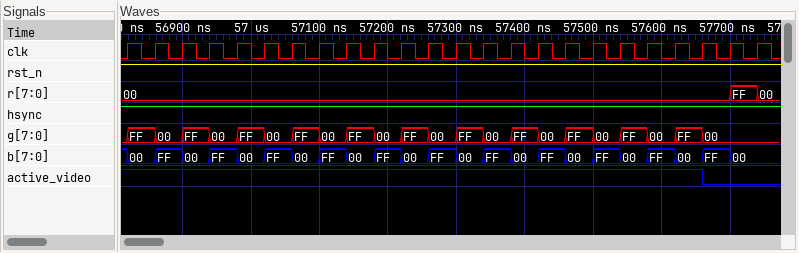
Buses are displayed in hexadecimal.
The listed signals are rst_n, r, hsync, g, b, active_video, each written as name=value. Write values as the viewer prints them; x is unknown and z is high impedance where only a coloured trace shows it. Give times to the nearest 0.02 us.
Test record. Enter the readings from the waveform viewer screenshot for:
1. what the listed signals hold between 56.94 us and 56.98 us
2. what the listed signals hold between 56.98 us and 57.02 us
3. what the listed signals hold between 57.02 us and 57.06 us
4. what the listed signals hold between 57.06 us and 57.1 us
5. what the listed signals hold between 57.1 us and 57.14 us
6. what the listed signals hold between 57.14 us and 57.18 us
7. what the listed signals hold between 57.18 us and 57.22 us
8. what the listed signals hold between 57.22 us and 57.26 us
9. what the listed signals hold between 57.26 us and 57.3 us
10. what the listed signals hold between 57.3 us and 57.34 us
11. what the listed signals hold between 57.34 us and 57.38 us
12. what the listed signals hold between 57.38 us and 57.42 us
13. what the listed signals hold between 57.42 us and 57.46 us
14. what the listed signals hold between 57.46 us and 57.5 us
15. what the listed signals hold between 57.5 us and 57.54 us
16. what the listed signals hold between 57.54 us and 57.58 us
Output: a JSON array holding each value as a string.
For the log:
["rst_n=1, r=00, hsync=1, g=00, b=FF, active_video=1", "rst_n=1, r=00, hsync=1, g=FF, b=00, active_video=1", "rst_n=1, r=00, hsync=1, g=00, b=FF, active_video=1", "rst_n=1, r=00, hsync=1, g=FF, b=00, active_video=1", "rst_n=1, r=00, hsync=1, g=00, b=FF, active_video=1", "rst_n=1, r=00, hsync=1, g=FF, b=00, active_video=1", "rst_n=1, r=00, hsync=1, g=00, b=FF, active_video=1", "rst_n=1, r=00, hsync=1, g=FF, b=00, active_video=1", "rst_n=1, r=00, hsync=1, g=00, b=FF, active_video=1", "rst_n=1, r=00, hsync=1, g=FF, b=00, active_video=1", "rst_n=1, r=00, hsync=1, g=00, b=FF, active_video=1", "rst_n=1, r=00, hsync=1, g=FF, b=00, active_video=1", "rst_n=1, r=00, hsync=1, g=00, b=FF, active_video=1", "rst_n=1, r=00, hsync=1, g=FF, b=00, active_video=1", "rst_n=1, r=00, hsync=1, g=00, b=FF, active_video=1", "rst_n=1, r=00, hsync=1, g=FF, b=00, active_video=1"]
